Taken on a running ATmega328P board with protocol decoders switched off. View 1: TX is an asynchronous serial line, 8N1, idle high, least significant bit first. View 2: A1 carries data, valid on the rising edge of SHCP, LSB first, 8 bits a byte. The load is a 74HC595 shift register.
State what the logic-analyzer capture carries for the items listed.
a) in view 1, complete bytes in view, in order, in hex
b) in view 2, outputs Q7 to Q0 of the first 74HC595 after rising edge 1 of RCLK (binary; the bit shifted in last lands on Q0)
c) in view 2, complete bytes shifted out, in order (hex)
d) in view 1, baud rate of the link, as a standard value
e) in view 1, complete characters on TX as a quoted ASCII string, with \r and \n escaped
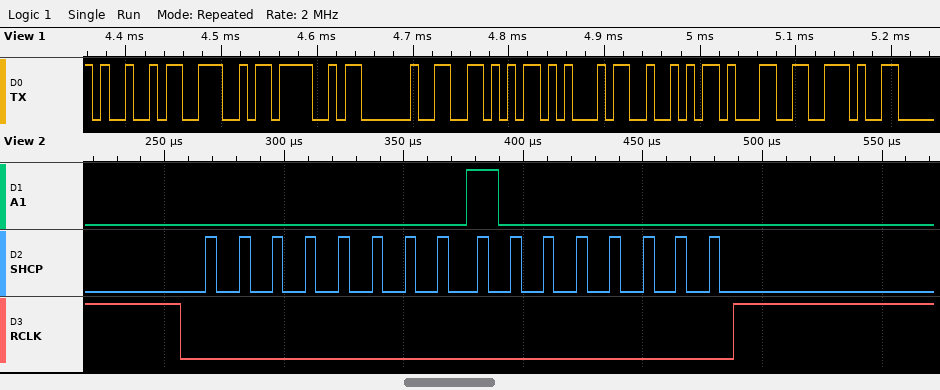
49 4E 4F 20 56 45 52 31 2E
10000000
00 01
115200 baud
"INO VER1."
